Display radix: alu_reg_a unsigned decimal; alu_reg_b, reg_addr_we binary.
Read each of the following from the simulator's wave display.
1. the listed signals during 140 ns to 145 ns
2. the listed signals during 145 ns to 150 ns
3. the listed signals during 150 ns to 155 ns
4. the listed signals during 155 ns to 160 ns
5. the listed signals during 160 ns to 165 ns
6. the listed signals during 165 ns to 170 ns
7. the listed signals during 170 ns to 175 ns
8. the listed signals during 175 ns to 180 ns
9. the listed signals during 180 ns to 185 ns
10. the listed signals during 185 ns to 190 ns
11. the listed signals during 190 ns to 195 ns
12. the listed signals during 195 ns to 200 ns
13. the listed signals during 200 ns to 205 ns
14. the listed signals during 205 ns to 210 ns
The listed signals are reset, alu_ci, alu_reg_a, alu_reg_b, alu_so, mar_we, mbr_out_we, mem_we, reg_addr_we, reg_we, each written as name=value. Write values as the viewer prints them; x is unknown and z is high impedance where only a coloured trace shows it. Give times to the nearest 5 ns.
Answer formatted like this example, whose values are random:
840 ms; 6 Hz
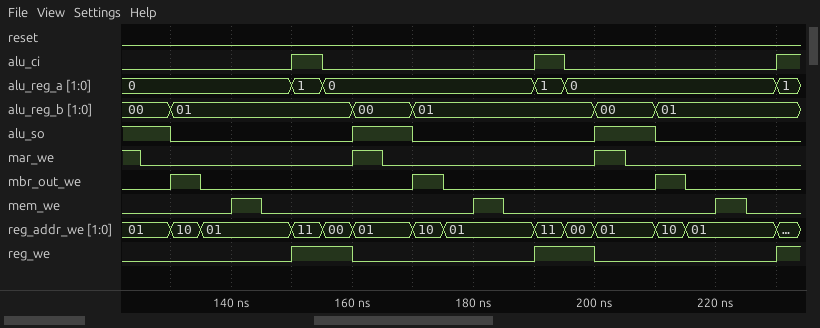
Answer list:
reset=0, alu_ci=0, alu_reg_a=0, alu_reg_b=01, alu_so=0, mar_we=0, mbr_out_we=0, mem_we=1, reg_addr_we=01, reg_we=0; reset=0, alu_ci=0, alu_reg_a=0, alu_reg_b=01, alu_so=0, mar_we=0, mbr_out_we=0, mem_we=0, reg_addr_we=01, reg_we=0; reset=0, alu_ci=1, alu_reg_a=1, alu_reg_b=01, alu_so=0, mar_we=0, mbr_out_we=0, mem_we=0, reg_addr_we=11, reg_we=1; reset=0, alu_ci=0, alu_reg_a=0, alu_reg_b=01, alu_so=0, mar_we=0, mbr_out_we=0, mem_we=0, reg_addr_we=00, reg_we=1; reset=0, alu_ci=0, alu_reg_a=0, alu_reg_b=00, alu_so=1, mar_we=1, mbr_out_we=0, mem_we=0, reg_addr_we=01, reg_we=0; reset=0, alu_ci=0, alu_reg_a=0, alu_reg_b=00, alu_so=1, mar_we=0, mbr_out_we=0, mem_we=0, reg_addr_we=01, reg_we=0; reset=0, alu_ci=0, alu_reg_a=0, alu_reg_b=01, alu_so=0, mar_we=0, mbr_out_we=1, mem_we=0, reg_addr_we=10, reg_we=0; reset=0, alu_ci=0, alu_reg_a=0, alu_reg_b=01, alu_so=0, mar_we=0, mbr_out_we=0, mem_we=0, reg_addr_we=01, reg_we=0; reset=0, alu_ci=0, alu_reg_a=0, alu_reg_b=01, alu_so=0, mar_we=0, mbr_out_we=0, mem_we=1, reg_addr_we=01, reg_we=0; reset=0, alu_ci=0, alu_reg_a=0, alu_reg_b=01, alu_so=0, mar_we=0, mbr_out_we=0, mem_we=0, reg_addr_we=01, reg_we=0; reset=0, alu_ci=1, alu_reg_a=1, alu_reg_b=01, alu_so=0, mar_we=0, mbr_out_we=0, mem_we=0, reg_addr_we=11, reg_we=1; reset=0, alu_ci=0, alu_reg_a=0, alu_reg_b=01, alu_so=0, mar_we=0, mbr_out_we=0, mem_we=0, reg_addr_we=00, reg_we=1; reset=0, alu_ci=0, alu_reg_a=0, alu_reg_b=00, alu_so=1, mar_we=1, mbr_out_we=0, mem_we=0, reg_addr_we=01, reg_we=0; reset=0, alu_ci=0, alu_reg_a=0, alu_reg_b=00, alu_so=1, mar_we=0, mbr_out_we=0, mem_we=0, reg_addr_we=01, reg_we=0
